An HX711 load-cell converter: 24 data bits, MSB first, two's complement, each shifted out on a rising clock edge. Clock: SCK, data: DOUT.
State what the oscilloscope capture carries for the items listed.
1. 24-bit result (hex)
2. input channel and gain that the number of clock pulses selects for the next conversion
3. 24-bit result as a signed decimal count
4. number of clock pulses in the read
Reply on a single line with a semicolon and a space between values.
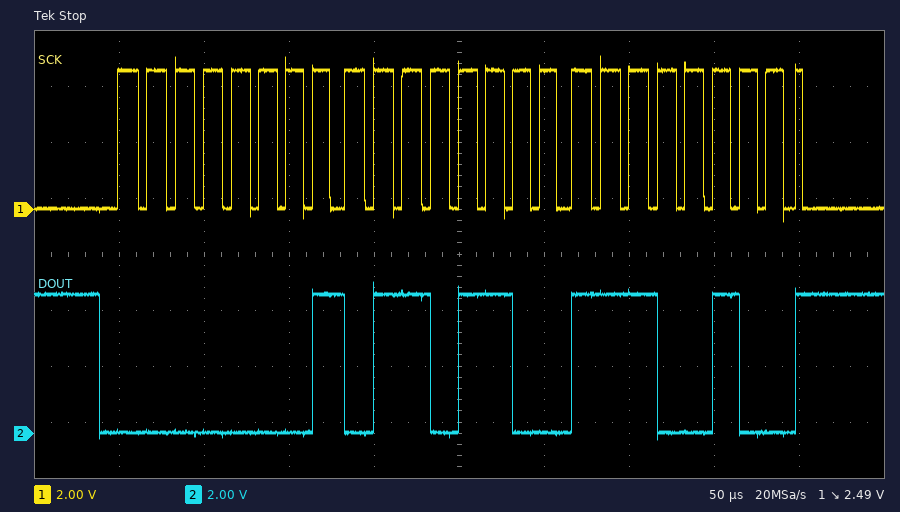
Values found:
0x016CE4; channel A, gain 128; 93412; 25
